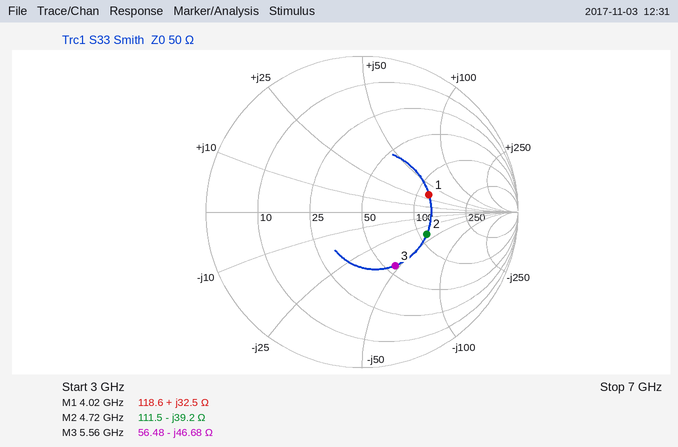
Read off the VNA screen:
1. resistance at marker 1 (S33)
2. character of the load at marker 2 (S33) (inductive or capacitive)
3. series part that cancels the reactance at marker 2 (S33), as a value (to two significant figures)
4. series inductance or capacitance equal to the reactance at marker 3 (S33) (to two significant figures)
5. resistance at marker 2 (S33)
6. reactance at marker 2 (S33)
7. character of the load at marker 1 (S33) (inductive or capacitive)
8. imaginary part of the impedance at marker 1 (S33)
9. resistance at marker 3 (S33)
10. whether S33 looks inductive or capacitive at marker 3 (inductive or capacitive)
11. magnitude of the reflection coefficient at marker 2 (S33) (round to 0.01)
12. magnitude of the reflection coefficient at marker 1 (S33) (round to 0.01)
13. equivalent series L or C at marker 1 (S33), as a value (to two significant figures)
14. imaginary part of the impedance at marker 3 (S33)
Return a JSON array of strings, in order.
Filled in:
["118.6 Ω", "capacitive", "1.3 nH", "610 fF", "111.5 Ω", "-39.2 Ω", "inductive", "+32.5 Ω", "56.48 Ω", "capacitive", "0.44", "0.44", "1.3 nH", "-46.68 Ω"]
